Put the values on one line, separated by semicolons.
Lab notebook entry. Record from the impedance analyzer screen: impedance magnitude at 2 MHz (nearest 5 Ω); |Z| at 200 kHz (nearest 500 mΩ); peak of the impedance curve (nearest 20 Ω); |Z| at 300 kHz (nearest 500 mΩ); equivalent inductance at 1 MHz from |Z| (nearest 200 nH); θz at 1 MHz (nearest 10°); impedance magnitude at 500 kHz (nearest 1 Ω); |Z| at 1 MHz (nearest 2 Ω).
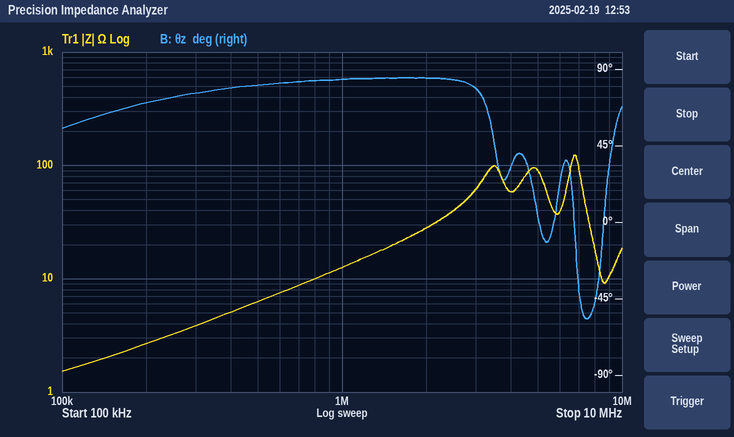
30 Ω; 2.5 Ω; 120 Ω; 4.0 Ω; 2.0 µH; 80°; 6 Ω; 12 Ω
